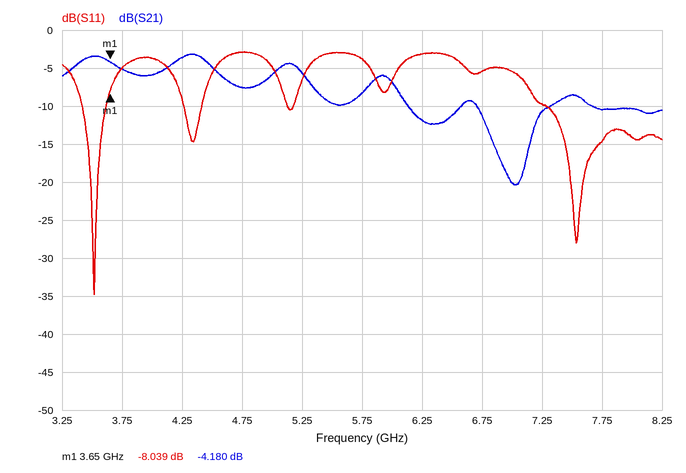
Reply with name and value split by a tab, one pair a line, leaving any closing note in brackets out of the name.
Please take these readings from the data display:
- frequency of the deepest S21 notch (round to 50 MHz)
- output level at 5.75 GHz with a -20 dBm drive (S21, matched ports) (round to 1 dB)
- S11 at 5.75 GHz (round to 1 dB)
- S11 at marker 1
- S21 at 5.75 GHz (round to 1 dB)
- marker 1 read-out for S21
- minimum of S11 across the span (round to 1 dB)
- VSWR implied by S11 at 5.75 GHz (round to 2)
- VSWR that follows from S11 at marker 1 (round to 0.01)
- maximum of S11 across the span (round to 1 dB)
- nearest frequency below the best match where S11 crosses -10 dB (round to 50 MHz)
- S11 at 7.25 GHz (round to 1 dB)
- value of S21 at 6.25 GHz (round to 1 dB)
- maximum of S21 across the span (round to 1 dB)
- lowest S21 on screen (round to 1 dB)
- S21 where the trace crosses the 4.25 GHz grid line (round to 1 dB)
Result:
frequency of the deepest S21 notch	7.00 GHz
output level at 5.75 GHz with a -20 dBm drive (S21, matched ports)	-28 dBm
S11 at 5.75 GHz	-4 dB
S11 at marker 1	-8.039 dB
S21 at 5.75 GHz	-8 dB
marker 1 read-out for S21	-4.180 dB
minimum of S11 across the span	-35 dB
VSWR implied by S11 at 5.75 GHz	4
VSWR that follows from S11 at marker 1	2.31
maximum of S11 across the span	-3 dB
nearest frequency below the best match where S11 crosses -10 dB	3.40 GHz
S11 at 7.25 GHz	-10 dB
value of S21 at 6.25 GHz	-12 dB
maximum of S21 across the span	-3 dB
lowest S21 on screen	-20 dB
S21 where the trace crosses the 4.25 GHz grid line	-4 dB
